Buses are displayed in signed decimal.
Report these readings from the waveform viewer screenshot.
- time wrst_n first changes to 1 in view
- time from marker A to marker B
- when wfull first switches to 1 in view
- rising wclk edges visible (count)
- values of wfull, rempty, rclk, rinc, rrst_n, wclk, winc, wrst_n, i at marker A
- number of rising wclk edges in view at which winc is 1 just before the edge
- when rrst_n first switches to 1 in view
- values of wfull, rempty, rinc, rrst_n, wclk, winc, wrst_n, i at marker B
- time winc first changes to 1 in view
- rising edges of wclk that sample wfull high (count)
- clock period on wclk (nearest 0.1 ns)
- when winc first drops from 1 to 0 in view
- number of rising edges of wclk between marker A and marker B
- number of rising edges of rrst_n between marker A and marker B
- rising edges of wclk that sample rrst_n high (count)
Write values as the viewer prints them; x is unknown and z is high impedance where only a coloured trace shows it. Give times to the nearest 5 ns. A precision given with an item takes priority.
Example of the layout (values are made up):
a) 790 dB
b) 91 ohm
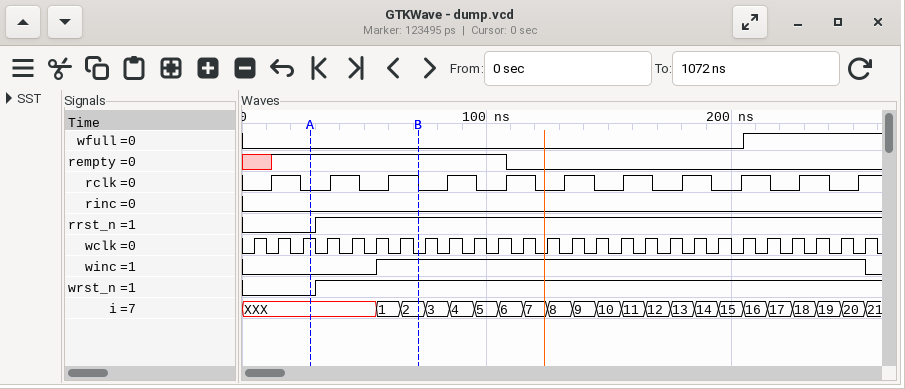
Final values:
a) 30 ns
b) 45 ns
c) 205 ns
d) 26
e) wfull=0, rempty=1, rclk=0, rinc=0, rrst_n=0, wclk=1, winc=0, wrst_n=0, i=XXX
f) 20
g) 30 ns
h) wfull=0, rempty=1, rinc=0, rrst_n=1, wclk=0, winc=1, wrst_n=1, i=2
i) 55 ns
j) 5
k) 10 ns
l) 255 ns
m) 4
n) 1
o) 23
